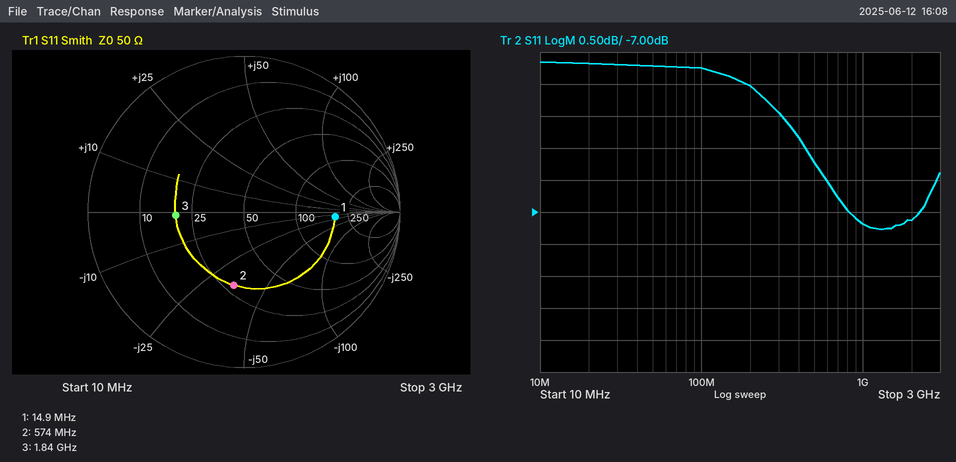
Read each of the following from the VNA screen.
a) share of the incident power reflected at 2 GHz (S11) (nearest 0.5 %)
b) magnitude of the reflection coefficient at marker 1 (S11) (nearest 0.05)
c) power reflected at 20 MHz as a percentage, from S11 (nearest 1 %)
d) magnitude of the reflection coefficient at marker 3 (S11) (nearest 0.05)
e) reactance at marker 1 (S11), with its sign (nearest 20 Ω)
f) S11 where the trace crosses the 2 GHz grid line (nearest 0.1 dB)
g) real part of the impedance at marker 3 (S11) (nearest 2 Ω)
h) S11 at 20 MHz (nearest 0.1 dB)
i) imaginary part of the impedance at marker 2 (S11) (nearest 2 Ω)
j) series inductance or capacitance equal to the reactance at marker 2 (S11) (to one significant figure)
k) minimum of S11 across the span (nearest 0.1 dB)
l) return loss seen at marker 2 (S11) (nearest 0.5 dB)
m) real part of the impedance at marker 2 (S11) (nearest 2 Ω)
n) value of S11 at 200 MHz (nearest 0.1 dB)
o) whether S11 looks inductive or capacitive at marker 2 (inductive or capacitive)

19.5 %
0.60
34 %
0.45
-20 Ω
-7.1 dB
20 Ω
-4.7 dB
-34 Ω
8 pF
-7.3 dB
6.5 dB
28 Ω
-5.0 dB
capacitive
